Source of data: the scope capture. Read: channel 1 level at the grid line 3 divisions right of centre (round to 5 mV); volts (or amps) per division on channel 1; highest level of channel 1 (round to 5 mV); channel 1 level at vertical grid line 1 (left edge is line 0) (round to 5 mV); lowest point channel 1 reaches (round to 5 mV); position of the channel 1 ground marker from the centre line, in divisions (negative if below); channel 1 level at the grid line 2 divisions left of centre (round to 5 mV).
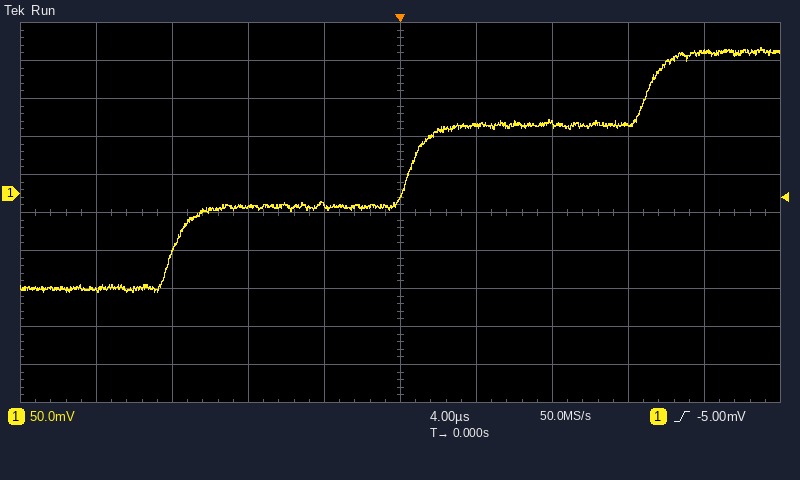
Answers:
90 mV
50 mV
190 mV
-125 mV
-130 mV
+0.5 div
-15 mV
